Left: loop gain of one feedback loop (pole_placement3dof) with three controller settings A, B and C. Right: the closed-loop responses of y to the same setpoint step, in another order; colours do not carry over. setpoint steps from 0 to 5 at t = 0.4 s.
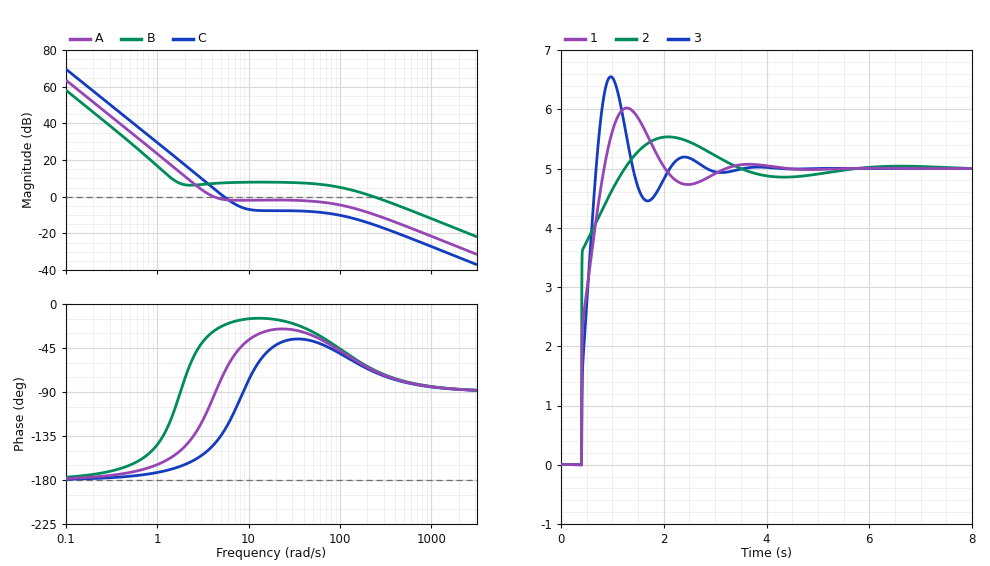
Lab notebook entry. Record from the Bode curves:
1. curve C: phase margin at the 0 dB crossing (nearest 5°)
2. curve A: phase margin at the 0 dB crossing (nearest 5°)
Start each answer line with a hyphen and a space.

- 50°
- 85°
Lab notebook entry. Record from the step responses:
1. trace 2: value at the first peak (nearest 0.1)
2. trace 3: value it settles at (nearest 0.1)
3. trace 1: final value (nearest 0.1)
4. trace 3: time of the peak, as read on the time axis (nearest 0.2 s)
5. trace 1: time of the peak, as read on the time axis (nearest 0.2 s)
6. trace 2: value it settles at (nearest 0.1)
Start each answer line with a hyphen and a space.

- 5.5
- 5.0
- 5.0
- 1.0 s
- 1.2 s
- 5.0
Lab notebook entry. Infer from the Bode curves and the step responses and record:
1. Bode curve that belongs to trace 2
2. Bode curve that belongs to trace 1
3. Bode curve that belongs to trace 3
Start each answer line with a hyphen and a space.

- B
- A
- C
